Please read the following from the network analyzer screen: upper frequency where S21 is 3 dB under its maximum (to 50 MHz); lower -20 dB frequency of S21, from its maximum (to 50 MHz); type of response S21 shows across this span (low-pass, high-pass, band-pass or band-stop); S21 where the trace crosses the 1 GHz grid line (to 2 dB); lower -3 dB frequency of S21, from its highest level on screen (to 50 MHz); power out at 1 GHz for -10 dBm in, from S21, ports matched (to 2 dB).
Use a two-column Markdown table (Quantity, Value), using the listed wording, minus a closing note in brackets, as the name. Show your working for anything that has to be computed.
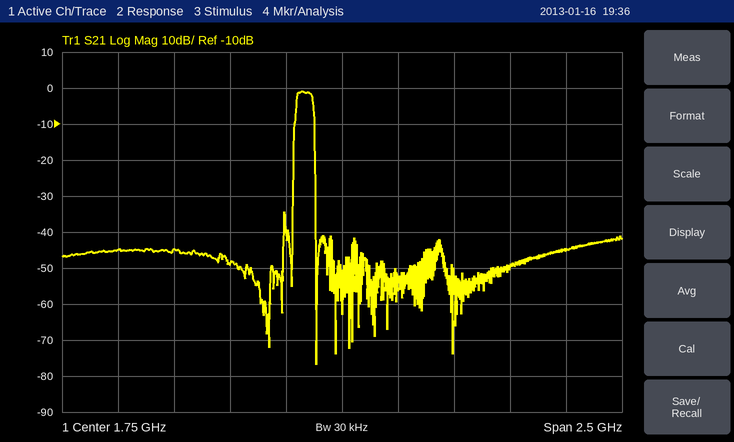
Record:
| Quantity | Value |
|---|---|
| upper frequency where S21 is 3 dB under its maximum | 1.60 GHz |
| lower -20 dB frequency of S21, from its maximum | 1.55 GHz |
| type of response S21 shows across this span | band-pass |
| S21 where the trace crosses the 1 GHz grid line | -44 dB |
| lower -3 dB frequency of S21, from its highest level on screen | 1.55 GHz |
| power out at 1 GHz for -10 dBm in, from S21, ports matched | -10 dBm + (-44 dB) = -54 dBm |
